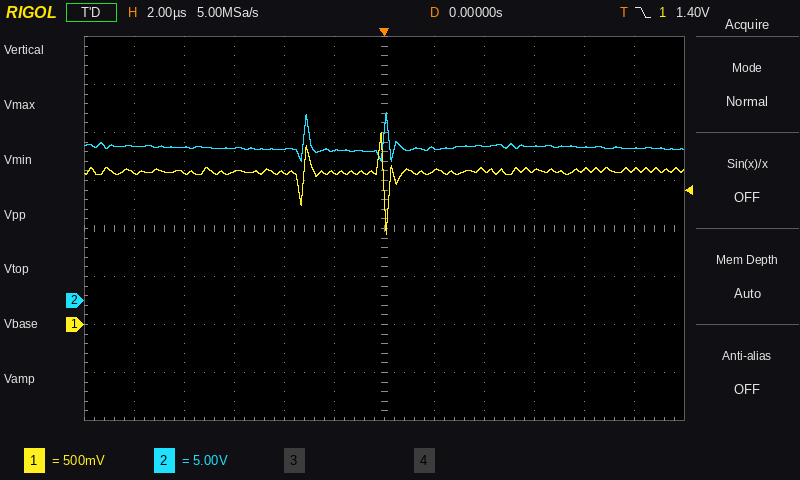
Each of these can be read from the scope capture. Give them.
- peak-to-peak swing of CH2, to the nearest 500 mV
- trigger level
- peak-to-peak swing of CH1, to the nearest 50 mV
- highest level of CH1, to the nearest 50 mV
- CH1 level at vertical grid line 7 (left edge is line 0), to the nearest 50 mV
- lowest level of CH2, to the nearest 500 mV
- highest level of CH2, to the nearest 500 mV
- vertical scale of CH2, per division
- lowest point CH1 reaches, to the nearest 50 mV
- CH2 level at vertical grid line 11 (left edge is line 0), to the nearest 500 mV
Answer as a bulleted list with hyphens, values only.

- 5.0 V
- 1.40 V
- 1.05 V
- 2.00 V
- 1.60 V
- 14.5 V
- 19.5 V
- 5 V
- 950 mV
- 16.0 V
